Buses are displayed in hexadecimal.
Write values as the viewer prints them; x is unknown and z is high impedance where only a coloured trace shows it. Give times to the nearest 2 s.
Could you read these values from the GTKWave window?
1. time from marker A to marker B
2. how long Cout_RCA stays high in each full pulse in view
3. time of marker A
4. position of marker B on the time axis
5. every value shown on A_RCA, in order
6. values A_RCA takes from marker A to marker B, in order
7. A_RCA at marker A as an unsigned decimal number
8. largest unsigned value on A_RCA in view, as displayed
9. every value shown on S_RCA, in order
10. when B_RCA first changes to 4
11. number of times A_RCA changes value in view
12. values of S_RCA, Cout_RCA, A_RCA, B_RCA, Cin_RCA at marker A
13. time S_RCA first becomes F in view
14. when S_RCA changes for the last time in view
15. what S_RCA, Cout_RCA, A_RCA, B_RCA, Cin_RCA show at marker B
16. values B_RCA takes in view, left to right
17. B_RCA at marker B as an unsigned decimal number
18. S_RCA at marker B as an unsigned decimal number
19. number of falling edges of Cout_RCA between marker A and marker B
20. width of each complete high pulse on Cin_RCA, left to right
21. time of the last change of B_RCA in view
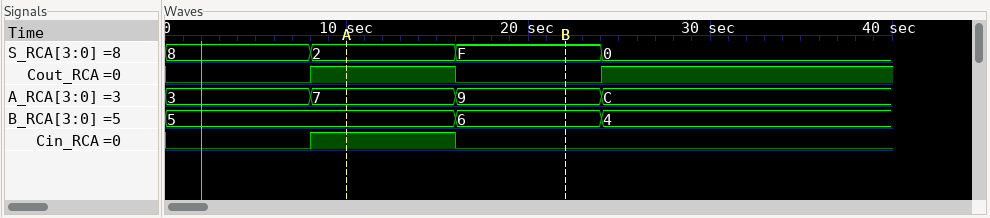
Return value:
12 s
8 s
10 s
22 s
3, 7, 9, C
7, 9
7
C
8, 2, F, 0
24 s
3
S_RCA=2, Cout_RCA=1, A_RCA=7, B_RCA=5, Cin_RCA=1
16 s
24 s
S_RCA=F, Cout_RCA=0, A_RCA=9, B_RCA=6, Cin_RCA=0
5, 6, 4
6
15
1
8 s
24 s
